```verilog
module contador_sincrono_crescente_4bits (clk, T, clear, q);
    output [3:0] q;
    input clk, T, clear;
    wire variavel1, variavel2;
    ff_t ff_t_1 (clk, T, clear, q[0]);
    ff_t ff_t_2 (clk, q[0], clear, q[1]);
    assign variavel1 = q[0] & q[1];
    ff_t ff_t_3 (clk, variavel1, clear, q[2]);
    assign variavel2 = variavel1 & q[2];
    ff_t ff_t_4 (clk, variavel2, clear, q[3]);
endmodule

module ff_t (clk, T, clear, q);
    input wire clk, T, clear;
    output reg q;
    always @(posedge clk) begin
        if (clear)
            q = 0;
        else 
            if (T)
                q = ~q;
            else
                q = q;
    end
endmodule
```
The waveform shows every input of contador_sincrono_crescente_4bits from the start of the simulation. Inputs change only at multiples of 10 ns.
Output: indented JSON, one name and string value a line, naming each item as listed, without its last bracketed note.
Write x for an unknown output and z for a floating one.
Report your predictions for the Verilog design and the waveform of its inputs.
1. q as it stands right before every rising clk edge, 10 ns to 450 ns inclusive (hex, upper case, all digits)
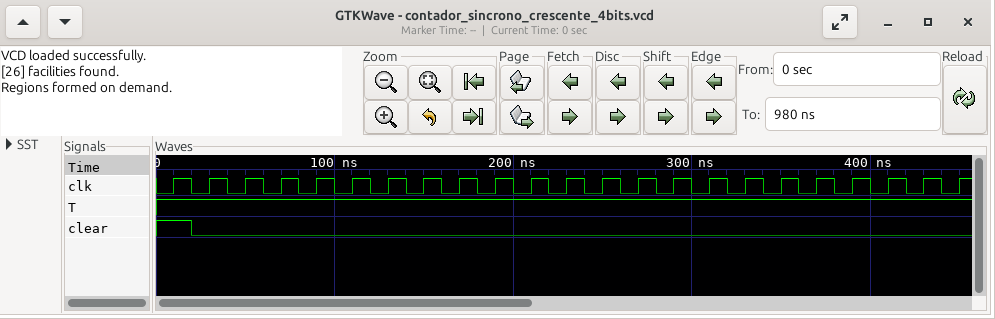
{
  "q as it stands right before every rising clk edge, 10 ns to 450 ns inclusive": "x, 0, 1, 2, 3, 4, 5, 6, 7, 8, 9, A, B, C, D, E, F, 0, 1, 2, 3, 4, 5"
}
